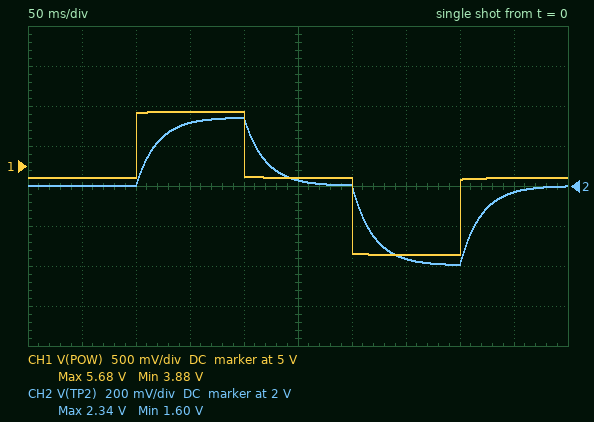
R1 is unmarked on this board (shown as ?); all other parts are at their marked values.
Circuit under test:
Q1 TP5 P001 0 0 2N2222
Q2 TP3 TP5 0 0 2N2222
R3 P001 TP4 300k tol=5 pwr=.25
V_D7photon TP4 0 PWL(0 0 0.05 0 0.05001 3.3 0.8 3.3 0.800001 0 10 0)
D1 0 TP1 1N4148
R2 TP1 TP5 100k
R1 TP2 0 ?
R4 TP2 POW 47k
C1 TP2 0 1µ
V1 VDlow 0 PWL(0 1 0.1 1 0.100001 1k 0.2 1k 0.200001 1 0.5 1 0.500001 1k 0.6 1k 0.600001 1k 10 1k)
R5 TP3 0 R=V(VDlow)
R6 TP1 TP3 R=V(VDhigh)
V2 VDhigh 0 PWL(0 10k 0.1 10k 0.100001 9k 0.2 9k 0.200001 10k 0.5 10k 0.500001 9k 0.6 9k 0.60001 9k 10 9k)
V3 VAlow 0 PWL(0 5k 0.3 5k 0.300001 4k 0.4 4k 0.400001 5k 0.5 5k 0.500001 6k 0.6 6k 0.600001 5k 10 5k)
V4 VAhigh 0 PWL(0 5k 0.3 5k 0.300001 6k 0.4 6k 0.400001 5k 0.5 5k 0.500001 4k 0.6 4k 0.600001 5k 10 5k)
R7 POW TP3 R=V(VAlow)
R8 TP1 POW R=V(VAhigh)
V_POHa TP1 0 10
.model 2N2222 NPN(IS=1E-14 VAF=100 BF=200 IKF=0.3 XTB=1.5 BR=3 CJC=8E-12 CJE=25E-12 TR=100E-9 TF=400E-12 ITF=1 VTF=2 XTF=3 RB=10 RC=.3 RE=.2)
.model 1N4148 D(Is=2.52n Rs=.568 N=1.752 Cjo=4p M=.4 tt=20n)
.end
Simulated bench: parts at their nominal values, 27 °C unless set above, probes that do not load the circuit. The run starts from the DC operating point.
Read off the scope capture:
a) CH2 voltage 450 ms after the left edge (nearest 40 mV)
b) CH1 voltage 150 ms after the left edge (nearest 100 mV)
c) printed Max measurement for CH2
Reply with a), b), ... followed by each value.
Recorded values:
a) 1.96 V
b) 5.7 V
c) 2.34 V
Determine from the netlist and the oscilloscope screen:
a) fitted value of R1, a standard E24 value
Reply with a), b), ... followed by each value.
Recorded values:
a) 33 kΩ
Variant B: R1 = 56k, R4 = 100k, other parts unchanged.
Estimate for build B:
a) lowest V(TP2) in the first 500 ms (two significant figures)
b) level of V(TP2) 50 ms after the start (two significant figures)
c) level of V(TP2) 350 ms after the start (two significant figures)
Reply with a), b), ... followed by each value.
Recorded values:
a) 1.4 V
b) 1.8 V
c) 1.5 V
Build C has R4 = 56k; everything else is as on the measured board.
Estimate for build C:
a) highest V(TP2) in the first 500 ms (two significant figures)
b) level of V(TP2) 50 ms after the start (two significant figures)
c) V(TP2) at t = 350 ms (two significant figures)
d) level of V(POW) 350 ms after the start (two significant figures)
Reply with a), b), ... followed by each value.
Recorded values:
a) 2.1 V
b) 1.8 V
c) 1.5 V
d) 3.9 V
